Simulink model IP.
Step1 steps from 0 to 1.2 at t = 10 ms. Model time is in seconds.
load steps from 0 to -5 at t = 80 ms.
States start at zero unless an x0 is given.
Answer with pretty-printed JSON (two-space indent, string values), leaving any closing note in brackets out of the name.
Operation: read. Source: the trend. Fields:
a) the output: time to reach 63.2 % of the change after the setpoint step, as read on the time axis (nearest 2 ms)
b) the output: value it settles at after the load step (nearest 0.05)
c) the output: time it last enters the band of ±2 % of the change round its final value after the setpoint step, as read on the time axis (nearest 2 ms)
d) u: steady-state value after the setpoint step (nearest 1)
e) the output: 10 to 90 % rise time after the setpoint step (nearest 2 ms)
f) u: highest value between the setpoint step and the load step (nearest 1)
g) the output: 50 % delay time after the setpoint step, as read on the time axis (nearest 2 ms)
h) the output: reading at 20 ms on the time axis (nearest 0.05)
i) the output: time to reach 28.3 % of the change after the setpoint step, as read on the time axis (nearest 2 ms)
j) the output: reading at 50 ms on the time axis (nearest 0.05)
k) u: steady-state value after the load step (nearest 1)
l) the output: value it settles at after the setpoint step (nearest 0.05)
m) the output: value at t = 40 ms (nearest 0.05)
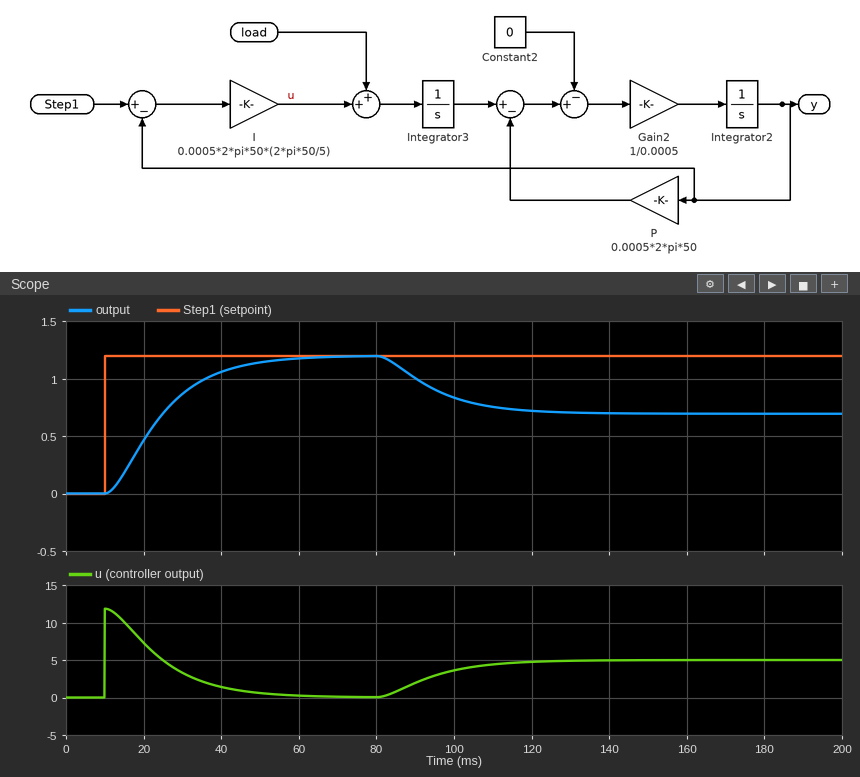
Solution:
{
  "the output: time to reach 63.2 % of the change after the setpoint step, as read on the time axis": "26 ms",
  "the output: value it settles at after the load step": "0.70",
  "the output: time it last enters the band of ±2 % of the change round its final value after the setpoint step, as read on the time axis": "60 ms",
  "u: steady-state value after the setpoint step": "0",
  "the output: 10 to 90 % rise time after the setpoint step": "28 ms",
  "u: highest value between the setpoint step and the load step": "12",
  "the output: 50 % delay time after the setpoint step, as read on the time axis": "22 ms",
  "the output: reading at 20 ms on the time axis": "0.45",
  "the output: time to reach 28.3 % of the change after the setpoint step, as read on the time axis": "18 ms",
  "the output: reading at 50 ms on the time axis": "1.15",
  "u: steady-state value after the load step": "5",
  "the output: value it settles at after the setpoint step": "1.20",
  "the output: value at t = 40 ms": "1.05"
}
